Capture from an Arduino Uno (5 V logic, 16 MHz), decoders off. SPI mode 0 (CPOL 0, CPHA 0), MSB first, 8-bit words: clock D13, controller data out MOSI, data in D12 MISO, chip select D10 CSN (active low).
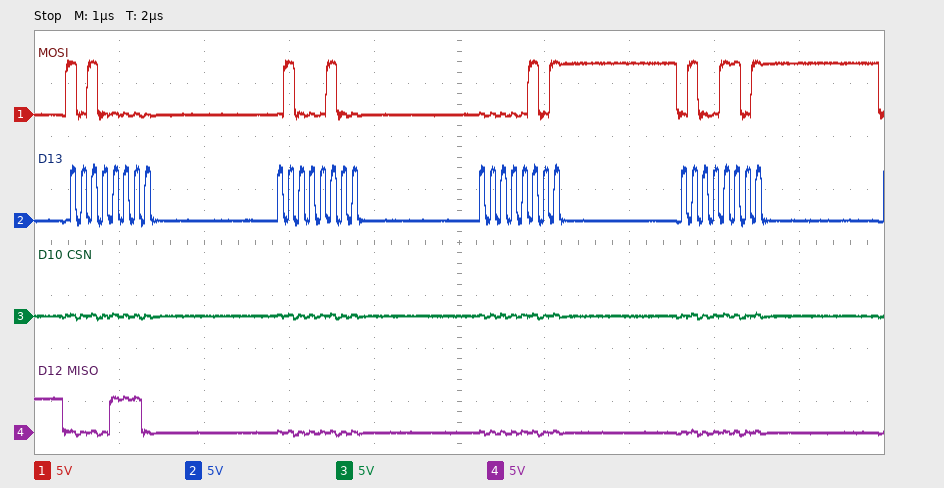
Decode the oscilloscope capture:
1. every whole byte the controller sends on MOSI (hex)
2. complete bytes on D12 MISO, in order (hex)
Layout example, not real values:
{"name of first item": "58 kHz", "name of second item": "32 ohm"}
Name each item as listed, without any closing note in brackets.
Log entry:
{"every whole byte the controller sends on MOSI": "A0 44 05 4D", "complete bytes on D12 MISO, in order": "0E 00 00 00"}
